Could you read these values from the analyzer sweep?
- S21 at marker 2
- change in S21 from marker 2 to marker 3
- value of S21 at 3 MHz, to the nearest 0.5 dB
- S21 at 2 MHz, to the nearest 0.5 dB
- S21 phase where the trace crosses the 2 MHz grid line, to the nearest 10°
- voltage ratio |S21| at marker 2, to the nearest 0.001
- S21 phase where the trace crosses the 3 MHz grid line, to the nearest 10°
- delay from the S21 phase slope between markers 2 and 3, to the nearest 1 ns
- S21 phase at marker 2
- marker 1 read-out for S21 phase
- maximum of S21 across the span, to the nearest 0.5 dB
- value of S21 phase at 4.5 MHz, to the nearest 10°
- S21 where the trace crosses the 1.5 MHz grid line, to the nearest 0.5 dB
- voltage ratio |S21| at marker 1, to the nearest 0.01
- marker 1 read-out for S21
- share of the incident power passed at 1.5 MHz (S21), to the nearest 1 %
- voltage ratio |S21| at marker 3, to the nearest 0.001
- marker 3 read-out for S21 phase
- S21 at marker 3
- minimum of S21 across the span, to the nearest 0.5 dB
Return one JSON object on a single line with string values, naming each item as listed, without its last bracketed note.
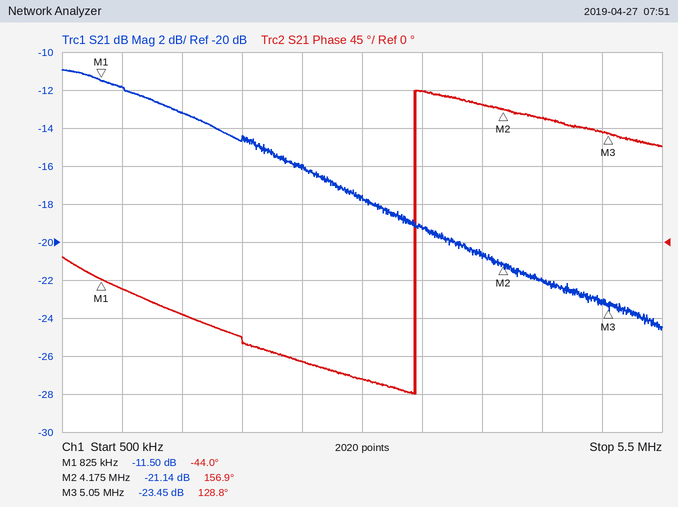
{"S21 at marker 2": "-21.14 dB", "change in S21 from marker 2 to marker 3": "-2.31 dB", "value of S21 at 3 MHz, to the nearest 0.5 dB": "-17.5 dB", "S21 at 2 MHz, to the nearest 0.5 dB": "-14.5 dB", "S21 phase where the trace crosses the 2 MHz grid line, to the nearest 10°": "-120°", "voltage ratio |S21| at marker 2, to the nearest 0.001": "0.088", "S21 phase where the trace crosses the 3 MHz grid line, to the nearest 10°": "-160°", "delay from the S21 phase slope between markers 2 and 3, to the nearest 1 ns": "89 ns", "S21 phase at marker 2": "156.9°", "marker 1 read-out for S21 phase": "-44.0°", "maximum of S21 across the span, to the nearest 0.5 dB": "-11.0 dB", "value of S21 phase at 4.5 MHz, to the nearest 10°": "150°", "S21 where the trace crosses the 1.5 MHz grid line, to the nearest 0.5 dB": "-13.0 dB", "voltage ratio |S21| at marker 1, to the nearest 0.01": "0.27", "marker 1 read-out for S21": "-11.50 dB", "share of the incident power passed at 1.5 MHz (S21), to the nearest 1 %": "5 %", "voltage ratio |S21| at marker 3, to the nearest 0.001": "0.067", "marker 3 read-out for S21 phase": "128.8°", "S21 at marker 3": "-23.45 dB", "minimum of S21 across the span, to the nearest 0.5 dB": "-24.5 dB"}
